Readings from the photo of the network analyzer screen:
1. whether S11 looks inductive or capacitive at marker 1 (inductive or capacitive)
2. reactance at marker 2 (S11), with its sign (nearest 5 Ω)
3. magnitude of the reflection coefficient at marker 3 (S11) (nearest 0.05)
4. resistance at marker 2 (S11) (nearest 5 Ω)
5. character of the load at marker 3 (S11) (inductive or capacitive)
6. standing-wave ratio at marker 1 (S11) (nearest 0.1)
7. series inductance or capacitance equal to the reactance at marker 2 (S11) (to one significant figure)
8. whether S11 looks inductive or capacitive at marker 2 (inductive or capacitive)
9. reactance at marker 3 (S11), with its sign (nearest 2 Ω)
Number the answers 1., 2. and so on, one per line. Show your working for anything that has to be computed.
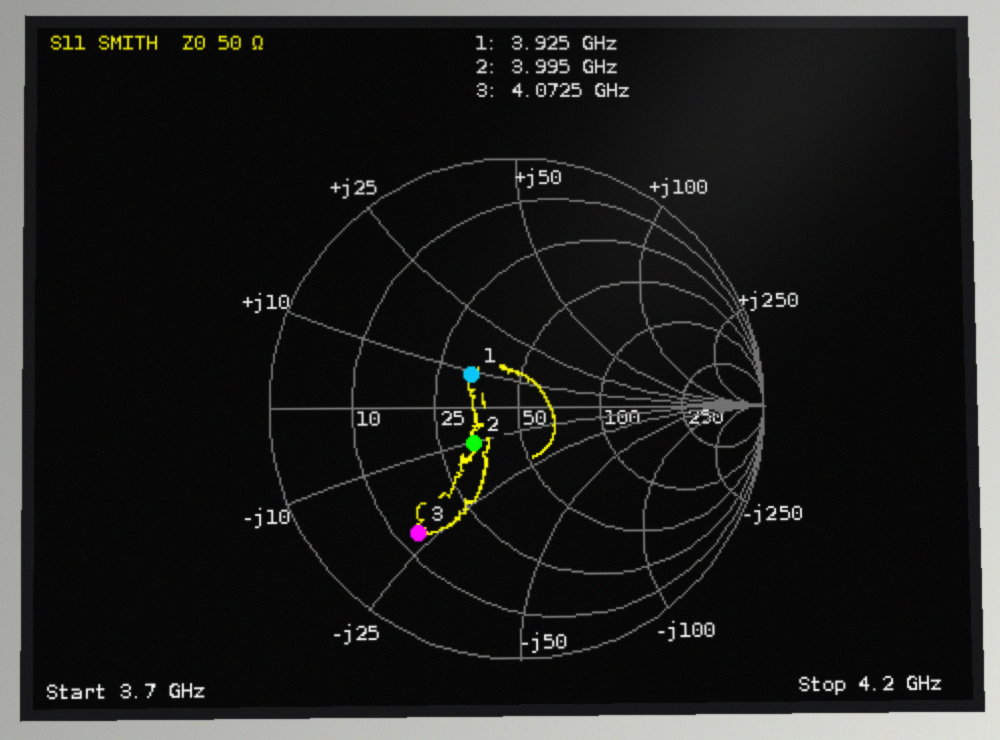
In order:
1. inductive
2. -10 Ω
3. 0.65
4. 35 Ω
5. capacitive
6. 1.6
7. C = 1/(2π × 3.995 GHz × 10 Ω) ≈ 4 pF
8. capacitive
9. -22 Ω
